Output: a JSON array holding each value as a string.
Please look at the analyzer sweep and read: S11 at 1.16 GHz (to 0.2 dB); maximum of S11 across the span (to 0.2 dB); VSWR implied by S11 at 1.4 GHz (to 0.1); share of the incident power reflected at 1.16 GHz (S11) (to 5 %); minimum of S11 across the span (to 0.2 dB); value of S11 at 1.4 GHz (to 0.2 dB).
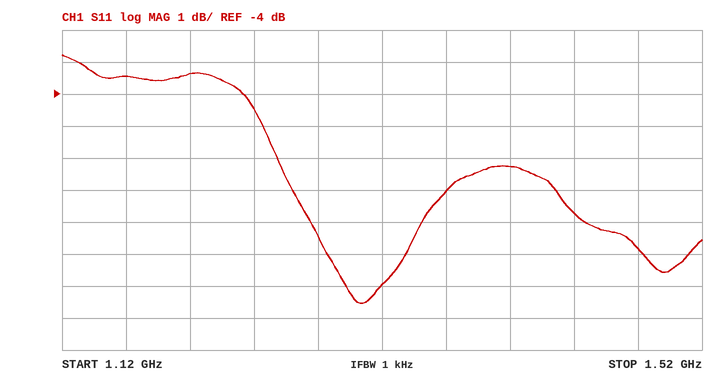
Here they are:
["-3.4 dB", "-2.8 dB", "2.9", "45 %", "-10.6 dB", "-6.2 dB"]
